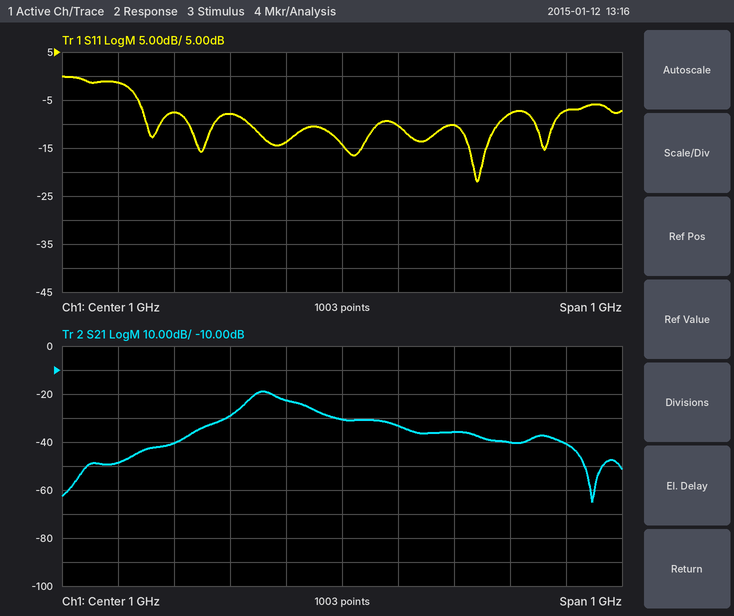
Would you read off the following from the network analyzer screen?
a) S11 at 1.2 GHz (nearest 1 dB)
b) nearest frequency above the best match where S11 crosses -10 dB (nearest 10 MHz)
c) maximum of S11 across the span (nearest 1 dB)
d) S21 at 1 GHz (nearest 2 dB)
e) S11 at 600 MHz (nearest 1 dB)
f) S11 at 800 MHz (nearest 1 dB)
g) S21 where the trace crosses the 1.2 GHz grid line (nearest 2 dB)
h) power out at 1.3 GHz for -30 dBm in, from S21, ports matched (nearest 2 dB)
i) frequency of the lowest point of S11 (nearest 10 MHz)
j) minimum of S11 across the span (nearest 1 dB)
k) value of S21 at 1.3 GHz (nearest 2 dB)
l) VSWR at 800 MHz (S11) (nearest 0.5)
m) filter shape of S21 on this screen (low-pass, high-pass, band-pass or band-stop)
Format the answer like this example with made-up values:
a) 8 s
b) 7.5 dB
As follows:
a) -10 dB
b) 1.28 GHz
c) 0 dB
d) -30 dB
e) -1 dB
f) -8 dB
g) -36 dB
h) -70 dBm
i) 1.24 GHz
j) -22 dB
k) -40 dB
l) 2.5
m) band-pass
